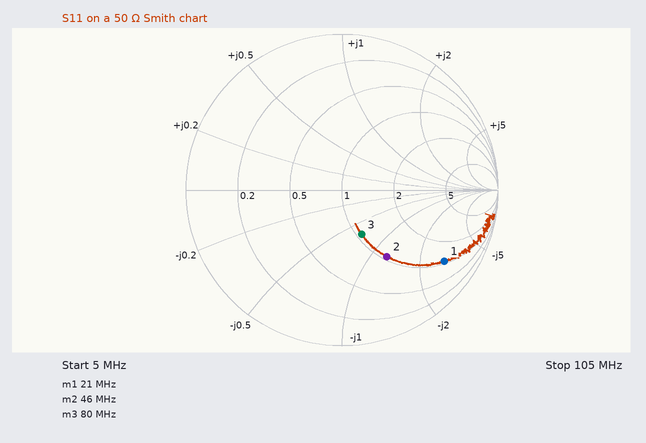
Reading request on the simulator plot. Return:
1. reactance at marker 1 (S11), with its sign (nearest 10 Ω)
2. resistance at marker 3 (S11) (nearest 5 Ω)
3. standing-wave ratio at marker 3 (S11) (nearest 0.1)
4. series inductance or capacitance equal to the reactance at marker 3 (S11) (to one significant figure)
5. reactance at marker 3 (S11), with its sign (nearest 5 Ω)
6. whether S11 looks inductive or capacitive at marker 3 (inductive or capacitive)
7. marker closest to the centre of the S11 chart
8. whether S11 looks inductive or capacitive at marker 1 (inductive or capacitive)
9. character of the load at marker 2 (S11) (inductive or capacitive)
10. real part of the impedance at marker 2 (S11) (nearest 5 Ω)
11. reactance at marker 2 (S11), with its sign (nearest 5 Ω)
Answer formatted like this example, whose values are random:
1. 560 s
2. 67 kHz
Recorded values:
1. -140 Ω
2. 55 Ω
3. 1.9
4. 60 pF
5. -35 Ω
6. capacitive
7. marker 3
8. capacitive
9. capacitive
10. 55 Ω
11. -60 Ω
